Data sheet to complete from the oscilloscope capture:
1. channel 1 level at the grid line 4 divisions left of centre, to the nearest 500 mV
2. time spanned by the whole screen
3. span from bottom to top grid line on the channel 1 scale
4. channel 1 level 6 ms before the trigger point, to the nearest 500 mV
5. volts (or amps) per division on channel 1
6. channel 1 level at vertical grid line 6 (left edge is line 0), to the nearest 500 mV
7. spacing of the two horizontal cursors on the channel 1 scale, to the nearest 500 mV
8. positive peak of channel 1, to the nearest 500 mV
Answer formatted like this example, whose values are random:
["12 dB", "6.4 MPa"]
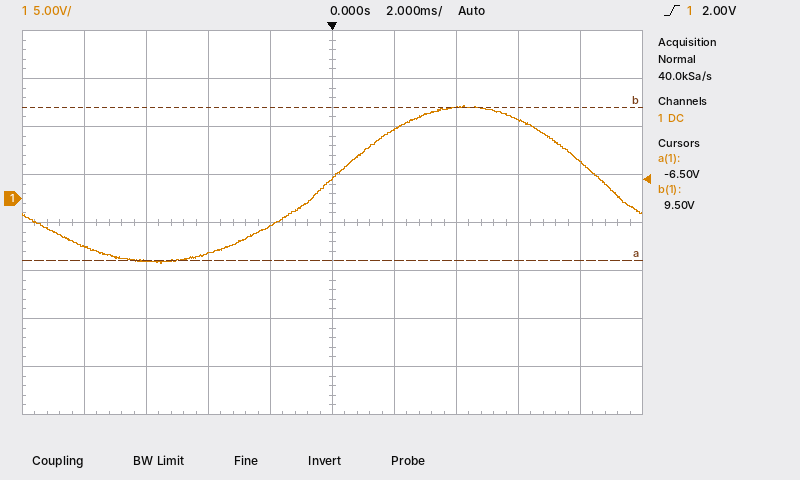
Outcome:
["-5.0 V", "20 ms", "40 V", "-6.5 V", "5 V", "7.0 V", "16.0 V", "9.5 V"]
